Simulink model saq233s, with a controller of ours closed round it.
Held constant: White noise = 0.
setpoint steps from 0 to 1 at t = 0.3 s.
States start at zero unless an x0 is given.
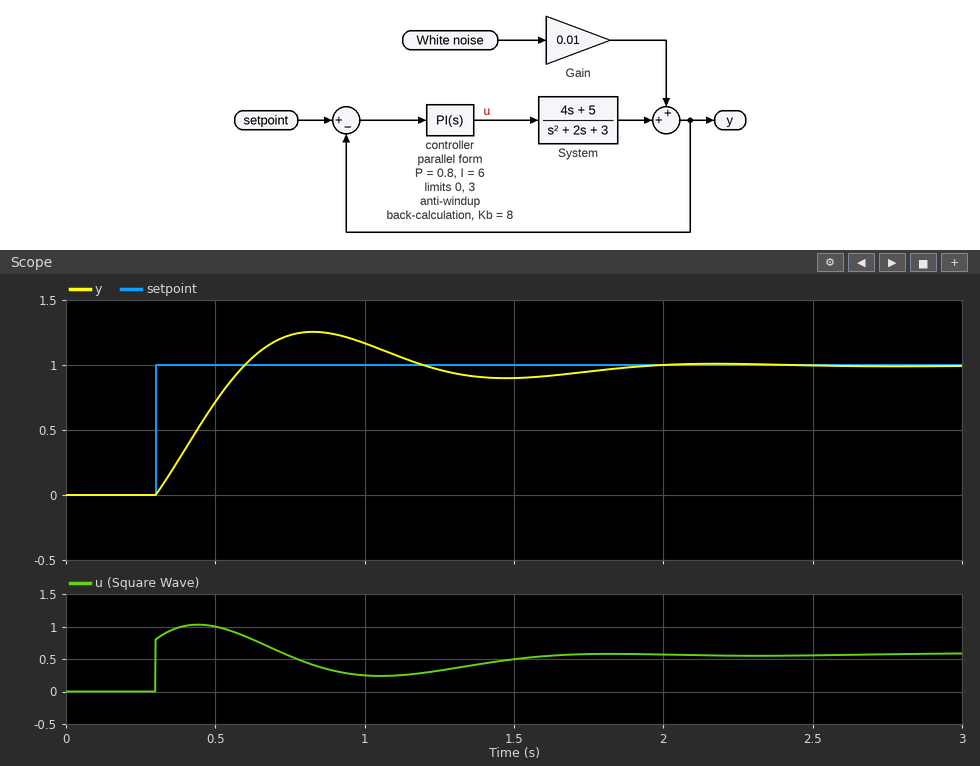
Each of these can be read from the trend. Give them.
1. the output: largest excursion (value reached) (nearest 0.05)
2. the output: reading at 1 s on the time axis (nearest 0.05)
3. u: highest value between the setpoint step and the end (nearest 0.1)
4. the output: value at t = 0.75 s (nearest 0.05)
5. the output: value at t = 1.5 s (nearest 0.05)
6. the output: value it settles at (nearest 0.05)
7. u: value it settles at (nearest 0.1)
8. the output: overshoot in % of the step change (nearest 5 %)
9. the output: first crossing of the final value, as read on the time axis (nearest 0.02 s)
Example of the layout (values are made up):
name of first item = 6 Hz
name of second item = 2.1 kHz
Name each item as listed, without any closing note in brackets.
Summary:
the output: largest excursion (value reached) = 1.25
the output: reading at 1 s on the time axis = 1.15
u: highest value between the setpoint step and the end = 1.0
the output: value at t = 0.75 s = 1.25
the output: value at t = 1.5 s = 0.90
the output: value it settles at = 1.00
u: value it settles at = 0.6
the output: overshoot in % of the step change = 25 %
the output: first crossing of the final value, as read on the time axis = 0.60 s
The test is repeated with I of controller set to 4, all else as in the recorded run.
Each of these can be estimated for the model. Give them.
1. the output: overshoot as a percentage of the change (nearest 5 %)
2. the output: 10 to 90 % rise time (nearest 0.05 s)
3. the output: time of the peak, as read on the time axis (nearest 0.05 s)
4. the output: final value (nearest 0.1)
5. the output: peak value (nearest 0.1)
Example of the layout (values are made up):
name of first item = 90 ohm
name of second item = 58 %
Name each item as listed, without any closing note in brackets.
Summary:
the output: overshoot as a percentage of the change = 15 %
the output: 10 to 90 % rise time = 0.30 s
the output: time of the peak, as read on the time axis = 0.90 s
the output: final value = 1.0
the output: peak value = 1.2
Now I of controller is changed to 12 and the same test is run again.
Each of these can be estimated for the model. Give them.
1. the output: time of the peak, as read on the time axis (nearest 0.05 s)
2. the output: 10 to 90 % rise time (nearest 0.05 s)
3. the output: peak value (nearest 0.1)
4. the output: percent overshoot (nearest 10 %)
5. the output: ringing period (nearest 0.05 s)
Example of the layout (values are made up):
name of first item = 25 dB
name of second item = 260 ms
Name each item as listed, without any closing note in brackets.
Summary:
the output: time of the peak, as read on the time axis = 0.70 s
the output: 10 to 90 % rise time = 0.15 s
the output: peak value = 1.4
the output: percent overshoot = 40 %
the output: ringing period = 0.95 s
